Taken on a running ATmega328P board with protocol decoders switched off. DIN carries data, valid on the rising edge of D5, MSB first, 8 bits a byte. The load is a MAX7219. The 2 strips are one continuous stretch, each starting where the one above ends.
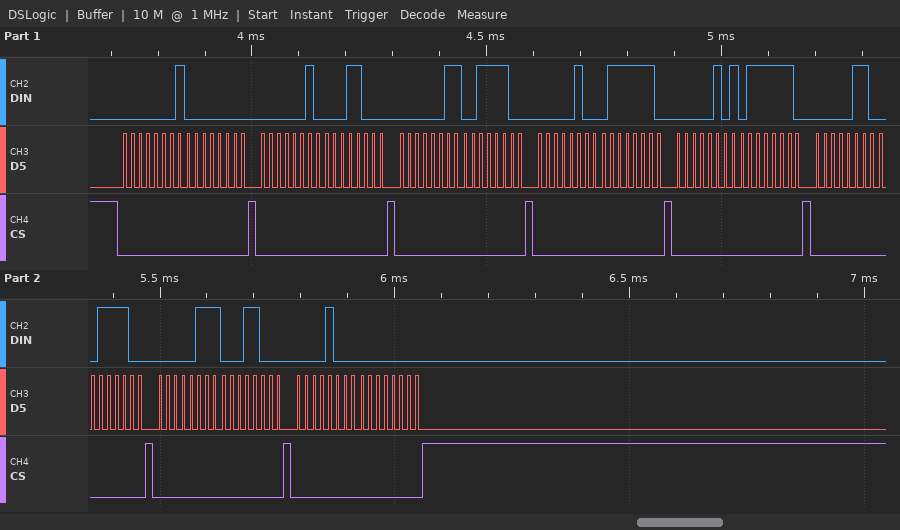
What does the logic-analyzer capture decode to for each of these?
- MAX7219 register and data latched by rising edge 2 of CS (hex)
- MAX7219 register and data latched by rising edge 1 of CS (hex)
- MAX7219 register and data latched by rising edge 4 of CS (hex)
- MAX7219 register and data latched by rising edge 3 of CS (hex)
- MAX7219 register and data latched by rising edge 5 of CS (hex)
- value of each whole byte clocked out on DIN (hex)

register 0x2, data 0x18
register 0x1, data 0x00
register 0x4, data 0x7E
register 0x3, data 0x3C
register 0x5, data 0x7E
01 00 02 18 03 3C 04 7E 05 7E 06 3C 07 18 08 00
